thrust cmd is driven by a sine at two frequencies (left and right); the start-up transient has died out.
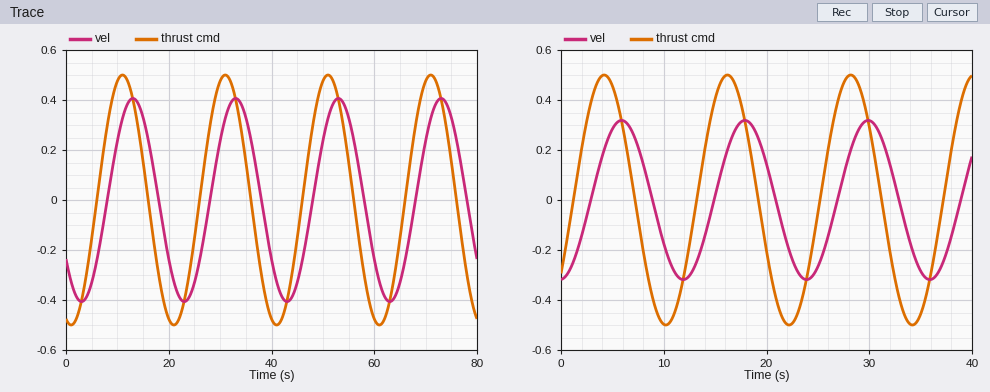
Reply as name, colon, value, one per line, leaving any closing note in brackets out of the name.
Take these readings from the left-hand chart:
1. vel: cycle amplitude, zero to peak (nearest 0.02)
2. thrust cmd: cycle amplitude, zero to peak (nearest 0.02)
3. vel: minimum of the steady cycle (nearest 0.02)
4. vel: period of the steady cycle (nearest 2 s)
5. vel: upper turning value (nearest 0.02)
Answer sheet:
vel: cycle amplitude, zero to peak: 0.40
thrust cmd: cycle amplitude, zero to peak: 0.50
vel: minimum of the steady cycle: -0.40
vel: period of the steady cycle: 20 s
vel: upper turning value: 0.40
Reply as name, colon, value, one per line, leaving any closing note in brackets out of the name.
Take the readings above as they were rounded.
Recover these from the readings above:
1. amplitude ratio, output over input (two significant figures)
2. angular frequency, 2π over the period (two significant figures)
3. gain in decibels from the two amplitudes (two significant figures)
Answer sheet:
amplitude ratio, output over input: 0.80
angular frequency, 2π over the period: 0.31 rad/s
gain in decibels from the two amplitudes: -1.9 dB
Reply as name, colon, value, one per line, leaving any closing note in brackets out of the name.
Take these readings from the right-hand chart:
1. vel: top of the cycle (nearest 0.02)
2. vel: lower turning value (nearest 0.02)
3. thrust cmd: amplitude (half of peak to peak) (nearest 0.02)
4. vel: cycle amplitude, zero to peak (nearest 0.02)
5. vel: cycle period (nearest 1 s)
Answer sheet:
vel: top of the cycle: 0.32
vel: lower turning value: -0.32
thrust cmd: amplitude (half of peak to peak): 0.50
vel: cycle amplitude, zero to peak: 0.32
vel: cycle period: 12 s
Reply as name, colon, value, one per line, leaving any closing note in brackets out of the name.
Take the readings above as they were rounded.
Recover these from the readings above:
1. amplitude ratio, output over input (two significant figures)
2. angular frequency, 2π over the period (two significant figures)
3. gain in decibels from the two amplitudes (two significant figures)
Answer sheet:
amplitude ratio, output over input: 0.64
angular frequency, 2π over the period: 0.52 rad/s
gain in decibels from the two amplitudes: -3.9 dB
